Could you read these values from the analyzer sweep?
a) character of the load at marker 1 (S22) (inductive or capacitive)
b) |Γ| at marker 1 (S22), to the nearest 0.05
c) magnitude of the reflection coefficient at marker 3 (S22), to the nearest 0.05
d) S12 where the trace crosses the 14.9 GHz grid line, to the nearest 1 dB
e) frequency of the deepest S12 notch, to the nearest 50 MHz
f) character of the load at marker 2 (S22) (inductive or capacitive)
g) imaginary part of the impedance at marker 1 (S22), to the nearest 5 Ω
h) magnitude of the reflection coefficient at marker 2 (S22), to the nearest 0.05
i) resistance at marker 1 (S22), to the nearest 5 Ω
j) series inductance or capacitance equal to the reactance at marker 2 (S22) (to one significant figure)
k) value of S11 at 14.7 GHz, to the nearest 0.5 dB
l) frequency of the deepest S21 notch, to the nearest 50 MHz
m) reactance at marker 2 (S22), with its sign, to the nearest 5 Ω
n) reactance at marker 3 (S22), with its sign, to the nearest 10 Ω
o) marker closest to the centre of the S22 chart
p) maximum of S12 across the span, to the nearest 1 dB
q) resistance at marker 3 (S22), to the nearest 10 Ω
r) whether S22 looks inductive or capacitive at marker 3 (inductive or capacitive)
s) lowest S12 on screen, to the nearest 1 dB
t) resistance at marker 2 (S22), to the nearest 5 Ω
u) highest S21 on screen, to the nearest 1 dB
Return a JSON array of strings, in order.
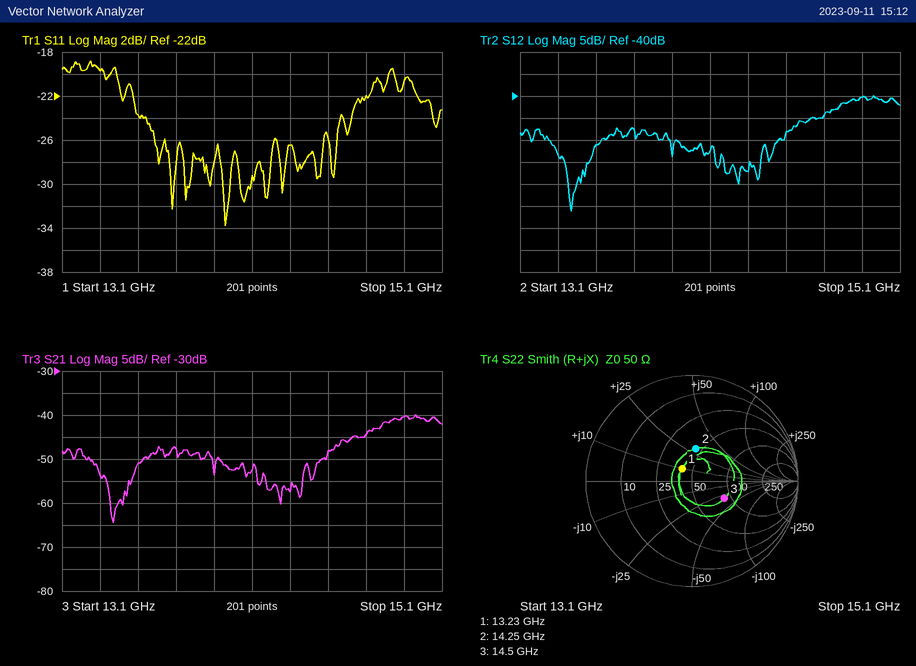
["inductive", "0.15", "0.35", "-40 dB", "13.35 GHz", "inductive", "+10 Ω", "0.30", "40 Ω", "300 pH", "-22.0 dB", "13.35 GHz", "+30 Ω", "-30 Ω", "marker 1", "-40 dB", "90 Ω", "capacitive", "-66 dB", "45 Ω", "-40 dB"]
